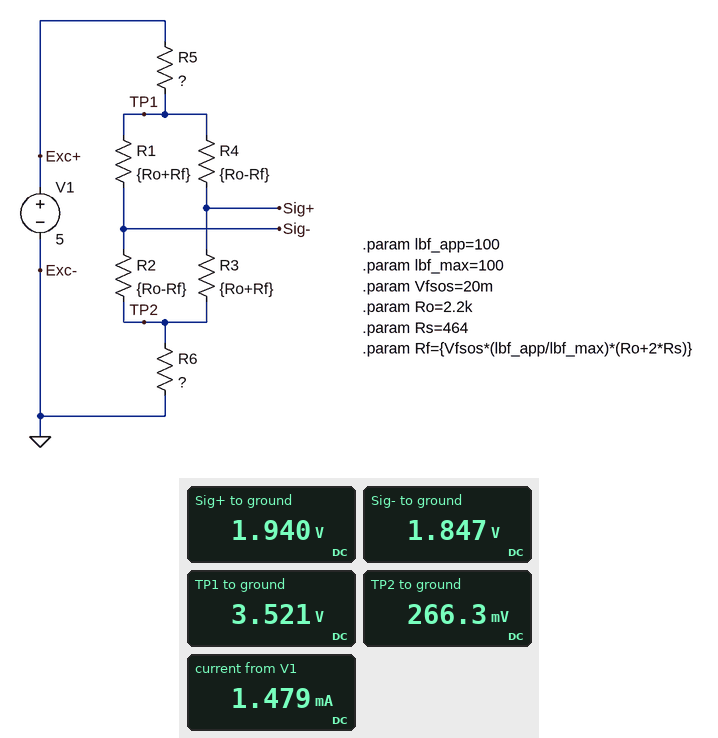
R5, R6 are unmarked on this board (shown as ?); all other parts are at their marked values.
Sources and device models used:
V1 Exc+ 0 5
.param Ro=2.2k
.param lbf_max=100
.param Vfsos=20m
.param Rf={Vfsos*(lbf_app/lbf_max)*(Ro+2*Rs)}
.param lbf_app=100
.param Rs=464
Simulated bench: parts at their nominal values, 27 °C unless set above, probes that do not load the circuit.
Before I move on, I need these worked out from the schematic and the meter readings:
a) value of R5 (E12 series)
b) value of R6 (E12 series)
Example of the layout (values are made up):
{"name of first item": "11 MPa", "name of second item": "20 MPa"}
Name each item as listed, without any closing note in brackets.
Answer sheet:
{"value of R5": "1 kΩ", "value of R6": "180 Ω"}
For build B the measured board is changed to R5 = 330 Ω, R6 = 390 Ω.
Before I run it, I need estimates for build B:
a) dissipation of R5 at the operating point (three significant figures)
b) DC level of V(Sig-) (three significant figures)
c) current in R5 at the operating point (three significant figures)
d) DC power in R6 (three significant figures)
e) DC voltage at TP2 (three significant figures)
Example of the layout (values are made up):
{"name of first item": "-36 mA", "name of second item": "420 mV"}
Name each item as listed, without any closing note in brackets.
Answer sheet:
{"dissipation of R5 at the operating point": "968 µW", "DC level of V(Sig-)": "2.50 V", "current in R5 at the operating point": "1.71 mA", "DC power in R6": "1.14 mW", "DC voltage at TP2": "668 mV"}
